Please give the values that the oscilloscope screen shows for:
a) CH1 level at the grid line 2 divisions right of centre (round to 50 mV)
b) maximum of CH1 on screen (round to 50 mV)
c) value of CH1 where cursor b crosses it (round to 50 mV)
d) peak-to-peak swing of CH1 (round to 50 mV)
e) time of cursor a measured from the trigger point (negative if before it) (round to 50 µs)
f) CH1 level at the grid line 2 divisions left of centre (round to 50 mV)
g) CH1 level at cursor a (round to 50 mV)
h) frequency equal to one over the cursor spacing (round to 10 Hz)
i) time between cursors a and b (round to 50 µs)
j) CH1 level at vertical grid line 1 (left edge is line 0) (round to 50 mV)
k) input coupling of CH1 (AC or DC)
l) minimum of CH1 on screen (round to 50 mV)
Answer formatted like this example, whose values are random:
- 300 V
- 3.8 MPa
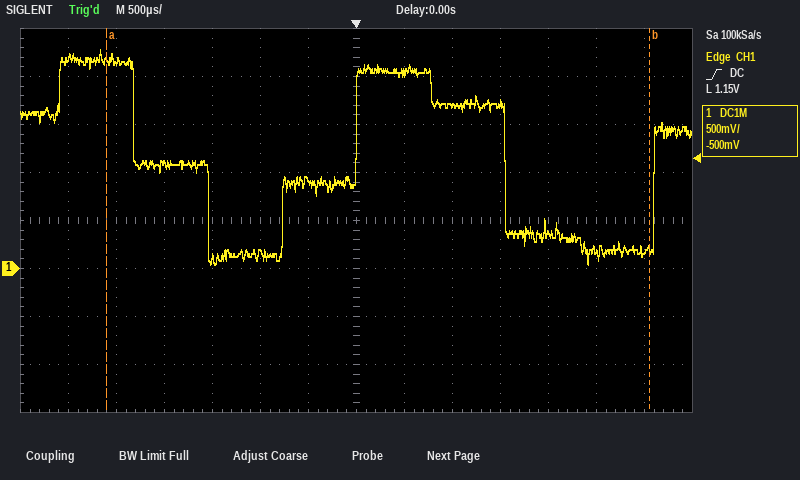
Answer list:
- 1.70 V
- 2.30 V
- 200 mV
- 2.25 V
- -2.60 ms
- 150 mV
- 2.15 V
- 180 Hz
- 5.65 ms
- 2.20 V
- DC
- 50 mV
